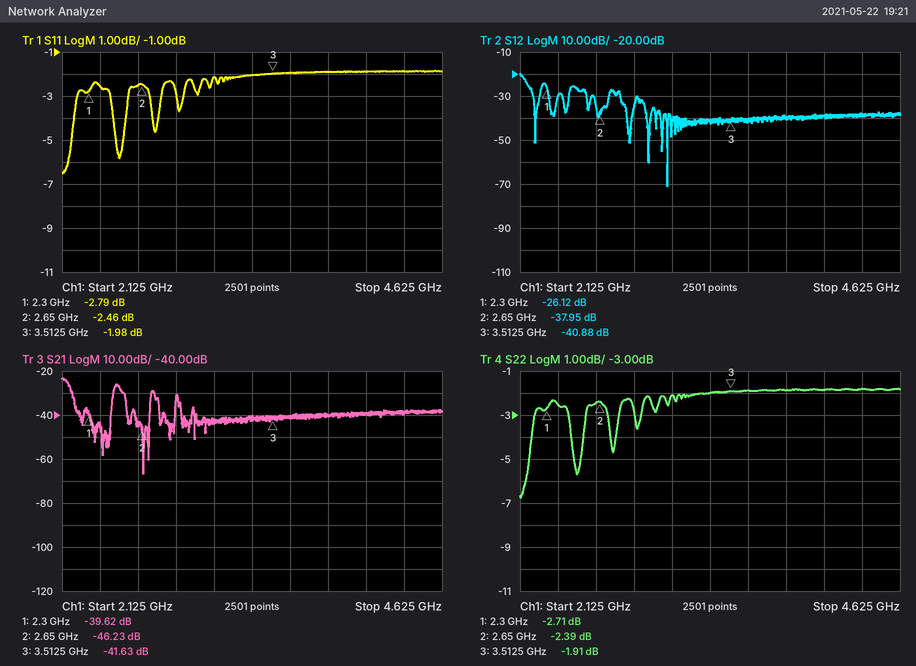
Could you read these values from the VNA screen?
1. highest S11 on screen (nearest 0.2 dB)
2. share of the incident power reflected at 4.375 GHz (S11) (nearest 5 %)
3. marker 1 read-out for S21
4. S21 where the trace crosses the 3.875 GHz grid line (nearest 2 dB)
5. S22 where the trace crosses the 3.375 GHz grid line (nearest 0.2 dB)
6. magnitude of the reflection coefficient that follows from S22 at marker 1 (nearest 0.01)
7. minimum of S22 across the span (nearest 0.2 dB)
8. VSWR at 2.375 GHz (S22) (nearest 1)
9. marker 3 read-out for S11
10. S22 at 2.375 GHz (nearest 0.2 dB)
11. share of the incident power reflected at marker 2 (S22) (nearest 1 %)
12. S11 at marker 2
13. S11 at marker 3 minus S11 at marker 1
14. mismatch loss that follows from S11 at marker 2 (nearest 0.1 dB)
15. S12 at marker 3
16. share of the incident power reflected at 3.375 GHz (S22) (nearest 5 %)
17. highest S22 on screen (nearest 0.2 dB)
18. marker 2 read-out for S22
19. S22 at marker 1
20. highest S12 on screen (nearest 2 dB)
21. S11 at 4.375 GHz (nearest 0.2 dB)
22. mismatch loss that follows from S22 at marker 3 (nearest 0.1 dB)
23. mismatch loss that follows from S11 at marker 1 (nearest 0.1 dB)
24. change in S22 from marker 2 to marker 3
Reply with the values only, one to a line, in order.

-1.8 dB
65 %
-39.62 dB
-40 dB
-2.0 dB
0.73
-6.8 dB
7
-1.98 dB
-2.6 dB
58 %
-2.46 dB
0.81 dB
3.6 dB
-40.88 dB
65 %
-1.8 dB
-2.39 dB
-2.71 dB
-20 dB
-1.8 dB
4.5 dB
3.2 dB
0.48 dB
